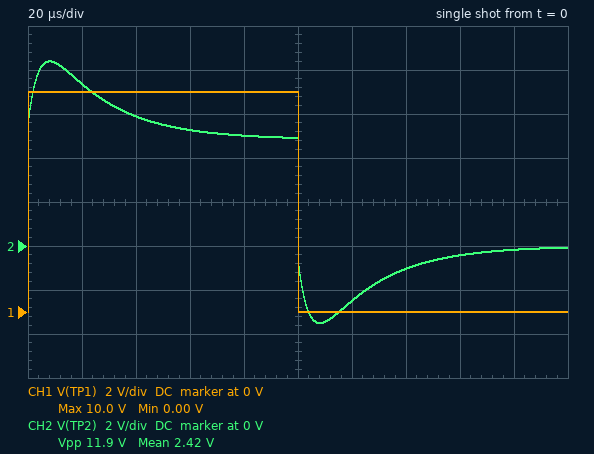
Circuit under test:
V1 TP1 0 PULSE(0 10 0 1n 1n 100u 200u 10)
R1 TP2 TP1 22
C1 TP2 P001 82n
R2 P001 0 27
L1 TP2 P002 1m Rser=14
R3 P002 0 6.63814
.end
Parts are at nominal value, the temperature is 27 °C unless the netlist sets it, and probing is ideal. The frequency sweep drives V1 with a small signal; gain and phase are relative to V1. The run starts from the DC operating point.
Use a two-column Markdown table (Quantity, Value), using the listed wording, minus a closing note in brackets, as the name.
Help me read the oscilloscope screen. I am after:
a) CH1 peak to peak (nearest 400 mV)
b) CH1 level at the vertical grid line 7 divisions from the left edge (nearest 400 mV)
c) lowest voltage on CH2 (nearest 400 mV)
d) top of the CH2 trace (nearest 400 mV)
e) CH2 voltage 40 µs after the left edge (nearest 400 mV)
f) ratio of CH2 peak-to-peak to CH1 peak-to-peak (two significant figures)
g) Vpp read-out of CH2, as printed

| Quantity | Value |
|---|---|
| CH1 peak to peak | 10.0 V |
| CH1 level at the vertical grid line 7 divisions from the left edge | 0 V |
| lowest voltage on CH2 | -3.6 V |
| top of the CH2 trace | 8.4 V |
| CH2 voltage 40 µs after the left edge | 6.0 V |
| ratio of CH2 peak-to-peak to CH1 peak-to-peak | 1.2 |
| Vpp read-out of CH2, as printed | 11.9 V |
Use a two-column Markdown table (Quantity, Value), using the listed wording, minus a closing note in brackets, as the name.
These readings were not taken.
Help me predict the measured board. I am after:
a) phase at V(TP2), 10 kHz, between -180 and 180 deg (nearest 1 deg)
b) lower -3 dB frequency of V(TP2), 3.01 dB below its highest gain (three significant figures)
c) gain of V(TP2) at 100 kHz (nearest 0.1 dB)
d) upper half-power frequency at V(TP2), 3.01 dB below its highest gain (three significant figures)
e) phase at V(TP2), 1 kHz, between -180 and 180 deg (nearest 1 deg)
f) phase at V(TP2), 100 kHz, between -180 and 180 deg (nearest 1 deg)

| Quantity | Value |
|---|---|
| phase at V(TP2), 10 kHz, between -180 and 180 deg | 10 deg |
| lower -3 dB frequency of V(TP2), 3.01 dB below its highest gain | 3.85 kHz |
| gain of V(TP2) at 100 kHz | -4.0 dB |
| upper half-power frequency at V(TP2), 3.01 dB below its highest gain | 87.2 kHz |
| phase at V(TP2), 1 kHz, between -180 and 180 deg | 8 deg |
| phase at V(TP2), 100 kHz, between -180 and 180 deg | -13 deg |
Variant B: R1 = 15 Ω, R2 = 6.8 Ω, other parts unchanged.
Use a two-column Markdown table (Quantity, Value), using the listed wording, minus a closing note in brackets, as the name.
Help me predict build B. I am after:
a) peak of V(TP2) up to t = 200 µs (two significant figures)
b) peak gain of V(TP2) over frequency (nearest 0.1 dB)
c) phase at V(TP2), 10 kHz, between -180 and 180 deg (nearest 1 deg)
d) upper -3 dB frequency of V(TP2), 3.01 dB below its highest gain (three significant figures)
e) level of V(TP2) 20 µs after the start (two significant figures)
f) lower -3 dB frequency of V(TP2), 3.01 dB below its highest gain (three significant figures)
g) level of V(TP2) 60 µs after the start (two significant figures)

| Quantity | Value |
|---|---|
| peak of V(TP2) up to t = 200 µs | 9.2 V |
| peak gain of V(TP2) over frequency | -0.3 dB |
| phase at V(TP2), 10 kHz, between -180 and 180 deg | 7 deg |
| upper -3 dB frequency of V(TP2), 3.01 dB below its highest gain | 108 kHz |
| level of V(TP2) 20 µs after the start | 8.0 V |
| lower -3 dB frequency of V(TP2), 3.01 dB below its highest gain | 2.83 kHz |
| level of V(TP2) 60 µs after the start | 6.3 V |
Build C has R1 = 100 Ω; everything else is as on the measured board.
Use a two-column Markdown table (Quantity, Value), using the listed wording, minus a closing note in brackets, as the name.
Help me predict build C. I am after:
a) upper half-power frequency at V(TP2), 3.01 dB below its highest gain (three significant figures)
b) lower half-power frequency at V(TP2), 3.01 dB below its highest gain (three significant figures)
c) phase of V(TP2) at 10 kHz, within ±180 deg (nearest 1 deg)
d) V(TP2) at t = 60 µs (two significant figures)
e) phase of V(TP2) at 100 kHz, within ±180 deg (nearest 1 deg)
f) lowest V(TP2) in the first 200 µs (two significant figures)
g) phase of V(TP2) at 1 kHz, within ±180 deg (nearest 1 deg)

| Quantity | Value |
|---|---|
| upper half-power frequency at V(TP2), 3.01 dB below its highest gain | 33.2 kHz |
| lower half-power frequency at V(TP2), 3.01 dB below its highest gain | 9.14 kHz |
| phase of V(TP2) at 10 kHz, within ±180 deg | 31 deg |
| V(TP2) at t = 60 µs | 1.6 V |
| phase of V(TP2) at 100 kHz, within ±180 deg | -25 deg |
| lowest V(TP2) in the first 200 µs | -3.4 V |
| phase of V(TP2) at 1 kHz, within ±180 deg | 13 deg |
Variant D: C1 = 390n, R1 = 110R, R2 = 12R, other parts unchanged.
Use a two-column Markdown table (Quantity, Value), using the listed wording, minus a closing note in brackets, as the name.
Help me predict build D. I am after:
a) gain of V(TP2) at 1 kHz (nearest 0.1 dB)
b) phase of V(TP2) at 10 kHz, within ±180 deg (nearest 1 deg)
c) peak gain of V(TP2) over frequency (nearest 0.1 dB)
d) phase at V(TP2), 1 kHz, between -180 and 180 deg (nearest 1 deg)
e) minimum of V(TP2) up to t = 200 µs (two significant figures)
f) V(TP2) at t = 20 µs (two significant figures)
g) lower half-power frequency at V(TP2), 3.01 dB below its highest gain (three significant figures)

| Quantity | Value |
|---|---|
| gain of V(TP2) at 1 kHz | -15.6 dB |
| phase of V(TP2) at 10 kHz, within ±180 deg | -22 deg |
| peak gain of V(TP2) over frequency | -7.1 dB |
| phase at V(TP2), 1 kHz, between -180 and 180 deg | 12 deg |
| minimum of V(TP2) up to t = 200 µs | -1.7 V |
| V(TP2) at t = 20 µs | 3.0 V |
| lower half-power frequency at V(TP2), 3.01 dB below its highest gain | 4.69 kHz |
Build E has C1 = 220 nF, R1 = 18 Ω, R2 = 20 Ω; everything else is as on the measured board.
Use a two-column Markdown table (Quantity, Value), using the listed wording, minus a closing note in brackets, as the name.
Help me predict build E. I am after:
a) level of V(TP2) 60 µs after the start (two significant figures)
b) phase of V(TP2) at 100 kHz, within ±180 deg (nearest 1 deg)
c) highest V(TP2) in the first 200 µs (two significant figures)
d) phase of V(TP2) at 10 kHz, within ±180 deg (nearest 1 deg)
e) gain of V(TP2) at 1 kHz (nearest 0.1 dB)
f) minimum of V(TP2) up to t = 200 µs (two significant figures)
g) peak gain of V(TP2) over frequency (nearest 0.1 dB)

| Quantity | Value |
|---|---|
| level of V(TP2) 60 µs after the start | 5.9 V |
| phase of V(TP2) at 100 kHz, within ±180 deg | -8 deg |
| highest V(TP2) in the first 200 µs | 7.9 V |
| phase of V(TP2) at 10 kHz, within ±180 deg | 1 deg |
| gain of V(TP2) at 1 kHz | -5.2 dB |
| minimum of V(TP2) up to t = 200 µs | -2.5 V |
| peak gain of V(TP2) over frequency | -1.2 dB |
